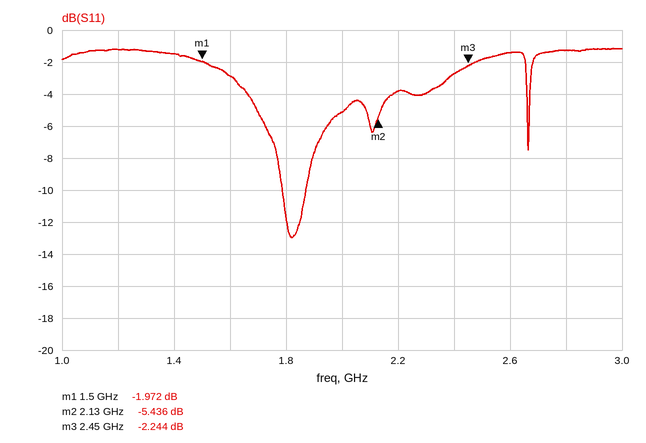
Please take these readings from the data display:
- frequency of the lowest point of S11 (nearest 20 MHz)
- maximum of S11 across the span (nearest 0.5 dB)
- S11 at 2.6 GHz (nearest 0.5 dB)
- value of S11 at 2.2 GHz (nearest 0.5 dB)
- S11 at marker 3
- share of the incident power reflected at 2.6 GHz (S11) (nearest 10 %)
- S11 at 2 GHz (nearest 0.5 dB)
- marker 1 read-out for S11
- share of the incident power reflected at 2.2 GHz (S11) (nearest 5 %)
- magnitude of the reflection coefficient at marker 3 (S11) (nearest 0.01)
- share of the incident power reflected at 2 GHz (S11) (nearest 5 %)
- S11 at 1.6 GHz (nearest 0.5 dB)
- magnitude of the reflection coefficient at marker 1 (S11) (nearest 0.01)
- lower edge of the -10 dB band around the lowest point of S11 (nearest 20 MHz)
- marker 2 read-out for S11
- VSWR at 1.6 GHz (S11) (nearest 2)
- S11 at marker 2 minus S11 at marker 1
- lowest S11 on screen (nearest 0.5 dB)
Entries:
1.82 GHz
-1.0 dB
-1.5 dB
-4.0 dB
-2.244 dB
70 %
-5.0 dB
-1.972 dB
40 %
0.77
30 %
-3.0 dB
0.80
1.78 GHz
-5.436 dB
6
-3.464 dB
-13.0 dB
